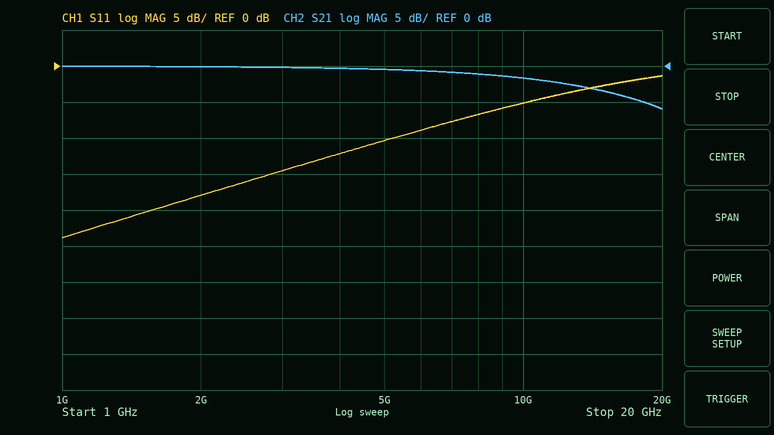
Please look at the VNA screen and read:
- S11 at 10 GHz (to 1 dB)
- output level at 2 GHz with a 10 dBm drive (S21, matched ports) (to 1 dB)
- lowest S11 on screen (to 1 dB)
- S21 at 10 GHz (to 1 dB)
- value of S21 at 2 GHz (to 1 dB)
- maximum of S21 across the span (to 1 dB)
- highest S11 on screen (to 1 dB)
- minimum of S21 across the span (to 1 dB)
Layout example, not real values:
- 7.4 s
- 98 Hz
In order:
- -5 dB
- 10 dBm
- -24 dB
- -2 dB
- 0 dB
- 0 dB
- -1 dB
- -6 dB
